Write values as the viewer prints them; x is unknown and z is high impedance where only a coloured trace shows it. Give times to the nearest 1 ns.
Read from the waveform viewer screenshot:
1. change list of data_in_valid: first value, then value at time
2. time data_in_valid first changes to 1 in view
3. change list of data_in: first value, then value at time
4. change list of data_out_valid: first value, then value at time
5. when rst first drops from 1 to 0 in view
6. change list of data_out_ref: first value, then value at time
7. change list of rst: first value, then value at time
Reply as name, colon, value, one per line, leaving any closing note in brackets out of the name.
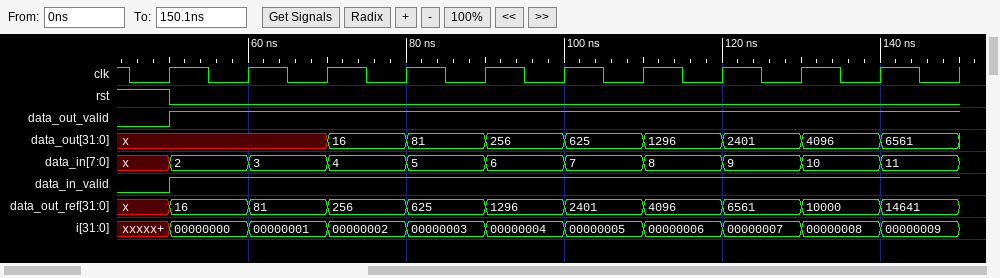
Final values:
change list of data_in_valid: first value, then value at time: 0, 1 at 50 ns
time data_in_valid first changes to 1 in view: 50 ns
change list of data_in: first value, then value at time: x, 2 at 50 ns, 3 at 60 ns, 4 at 70 ns, 5 at 80 ns, 6 at 90 ns, 7 at 100 ns, 8 at 110 ns, 9 at 120 ns, 10 at 130 ns, 11 at 140 ns
change list of data_out_valid: first value, then value at time: 0, 1 at 50 ns
when rst first drops from 1 to 0 in view: 50 ns
change list of data_out_ref: first value, then value at time: x, 16 at 50 ns, 81 at 60 ns, 256 at 70 ns, 625 at 80 ns, 1296 at 90 ns, 2401 at 100 ns, 4096 at 110 ns, 6561 at 120 ns, 10000 at 130 ns, 14641 at 140 ns
change list of rst: first value, then value at time: 1, 0 at 50 ns
